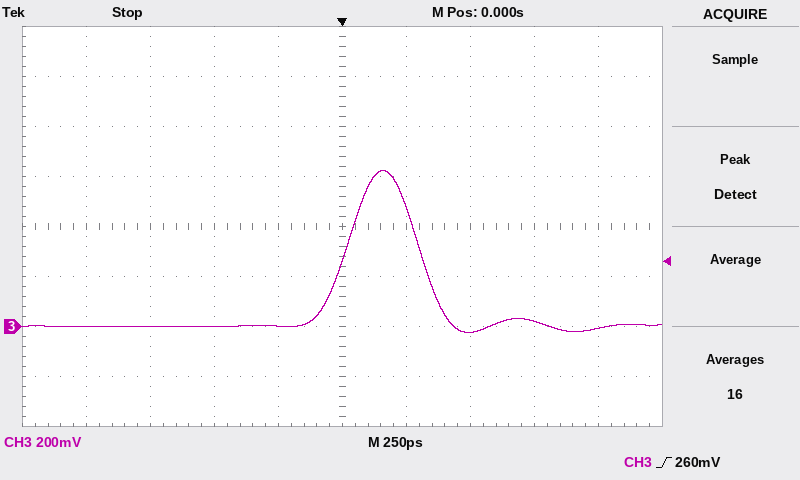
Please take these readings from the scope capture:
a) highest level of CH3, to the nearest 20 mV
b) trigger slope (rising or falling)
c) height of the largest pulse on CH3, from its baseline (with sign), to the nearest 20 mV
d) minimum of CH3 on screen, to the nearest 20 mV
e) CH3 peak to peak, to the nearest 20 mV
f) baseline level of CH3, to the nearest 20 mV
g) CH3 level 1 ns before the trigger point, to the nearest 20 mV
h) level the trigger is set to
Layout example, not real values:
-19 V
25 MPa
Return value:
620 mV
rising
+620 mV
-20 mV
640 mV
0 mV
0 mV
260 mV
